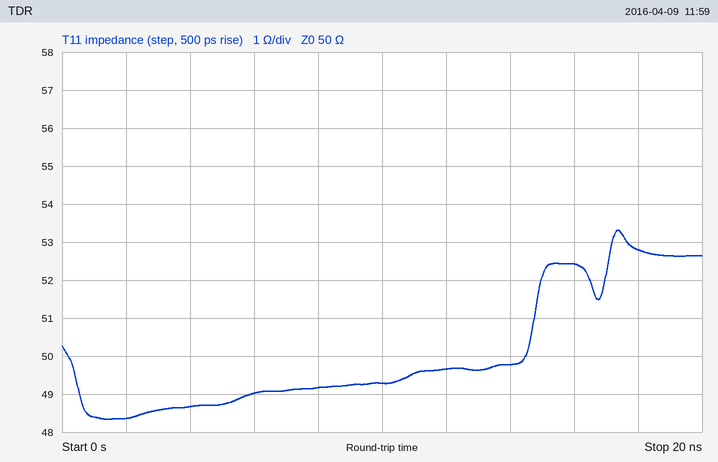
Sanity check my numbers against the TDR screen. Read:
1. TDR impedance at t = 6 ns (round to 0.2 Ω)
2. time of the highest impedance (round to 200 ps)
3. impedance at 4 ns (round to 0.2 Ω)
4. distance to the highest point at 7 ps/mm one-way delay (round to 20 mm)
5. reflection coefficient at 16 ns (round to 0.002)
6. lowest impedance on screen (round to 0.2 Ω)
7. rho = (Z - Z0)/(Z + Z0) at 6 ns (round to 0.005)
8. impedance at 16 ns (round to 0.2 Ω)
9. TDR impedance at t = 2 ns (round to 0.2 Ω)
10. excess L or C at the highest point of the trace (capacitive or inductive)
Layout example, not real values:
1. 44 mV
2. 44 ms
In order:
1. 49.0 Ω
2. 17.4 ns
3. 48.6 Ω
4. 1.24 m
5. +0.024
6. 48.4 Ω
7. -0.010
8. 52.4 Ω
9. 48.4 Ω
10. inductive
